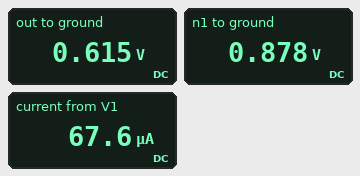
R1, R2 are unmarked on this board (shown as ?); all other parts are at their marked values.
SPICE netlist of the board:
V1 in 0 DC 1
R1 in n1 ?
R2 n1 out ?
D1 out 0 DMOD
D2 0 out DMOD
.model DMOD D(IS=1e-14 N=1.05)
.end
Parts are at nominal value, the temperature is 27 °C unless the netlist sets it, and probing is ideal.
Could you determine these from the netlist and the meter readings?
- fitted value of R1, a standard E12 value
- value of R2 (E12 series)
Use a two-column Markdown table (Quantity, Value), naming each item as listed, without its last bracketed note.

| Quantity | Value |
|---|---|
| fitted value of R1, a standard E12 value | 1.8 kΩ |
| value of R2 | 3.9 kΩ |
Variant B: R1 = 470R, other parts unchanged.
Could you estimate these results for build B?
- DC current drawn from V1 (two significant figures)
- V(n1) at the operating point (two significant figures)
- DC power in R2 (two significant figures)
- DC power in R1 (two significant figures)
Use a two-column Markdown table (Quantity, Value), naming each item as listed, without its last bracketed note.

| Quantity | Value |
|---|---|
| DC current drawn from V1 | 87 µA |
| V(n1) at the operating point | 960 mV |
| DC power in R2 | 29 µW |
| DC power in R1 | 3.5 µW |
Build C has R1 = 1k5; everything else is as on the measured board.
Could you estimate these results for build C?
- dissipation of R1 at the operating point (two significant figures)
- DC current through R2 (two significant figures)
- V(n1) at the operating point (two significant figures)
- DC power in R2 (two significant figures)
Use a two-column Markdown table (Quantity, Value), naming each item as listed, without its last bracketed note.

| Quantity | Value |
|---|---|
| dissipation of R1 at the operating point | 7.6 µW |
| DC current through R2 | 71 µA |
| V(n1) at the operating point | 890 mV |
| DC power in R2 | 20 µW |
